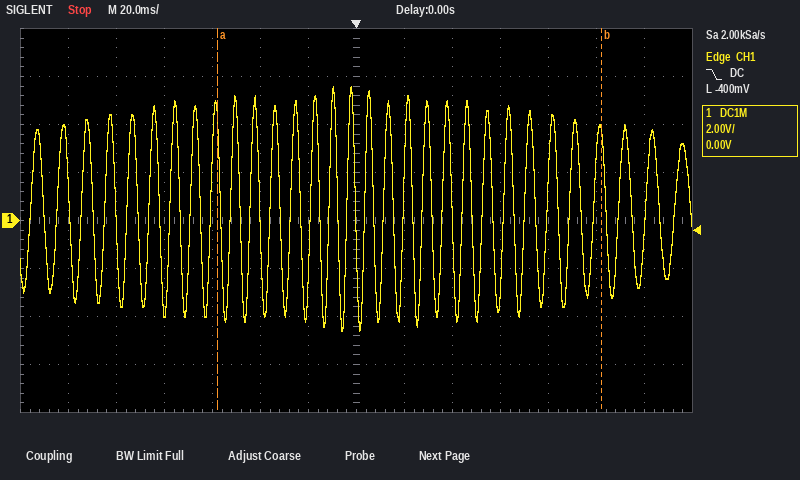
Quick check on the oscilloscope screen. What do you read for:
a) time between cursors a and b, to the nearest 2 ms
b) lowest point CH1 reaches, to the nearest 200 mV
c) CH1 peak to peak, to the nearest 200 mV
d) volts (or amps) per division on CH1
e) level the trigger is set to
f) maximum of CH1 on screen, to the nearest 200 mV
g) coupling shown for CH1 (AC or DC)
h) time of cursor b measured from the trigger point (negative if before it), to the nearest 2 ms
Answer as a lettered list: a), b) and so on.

a) 160 ms
b) -4.6 V
c) 10.2 V
d) 2 V
e) -400 mV
f) 5.6 V
g) DC
h) +102 ms
